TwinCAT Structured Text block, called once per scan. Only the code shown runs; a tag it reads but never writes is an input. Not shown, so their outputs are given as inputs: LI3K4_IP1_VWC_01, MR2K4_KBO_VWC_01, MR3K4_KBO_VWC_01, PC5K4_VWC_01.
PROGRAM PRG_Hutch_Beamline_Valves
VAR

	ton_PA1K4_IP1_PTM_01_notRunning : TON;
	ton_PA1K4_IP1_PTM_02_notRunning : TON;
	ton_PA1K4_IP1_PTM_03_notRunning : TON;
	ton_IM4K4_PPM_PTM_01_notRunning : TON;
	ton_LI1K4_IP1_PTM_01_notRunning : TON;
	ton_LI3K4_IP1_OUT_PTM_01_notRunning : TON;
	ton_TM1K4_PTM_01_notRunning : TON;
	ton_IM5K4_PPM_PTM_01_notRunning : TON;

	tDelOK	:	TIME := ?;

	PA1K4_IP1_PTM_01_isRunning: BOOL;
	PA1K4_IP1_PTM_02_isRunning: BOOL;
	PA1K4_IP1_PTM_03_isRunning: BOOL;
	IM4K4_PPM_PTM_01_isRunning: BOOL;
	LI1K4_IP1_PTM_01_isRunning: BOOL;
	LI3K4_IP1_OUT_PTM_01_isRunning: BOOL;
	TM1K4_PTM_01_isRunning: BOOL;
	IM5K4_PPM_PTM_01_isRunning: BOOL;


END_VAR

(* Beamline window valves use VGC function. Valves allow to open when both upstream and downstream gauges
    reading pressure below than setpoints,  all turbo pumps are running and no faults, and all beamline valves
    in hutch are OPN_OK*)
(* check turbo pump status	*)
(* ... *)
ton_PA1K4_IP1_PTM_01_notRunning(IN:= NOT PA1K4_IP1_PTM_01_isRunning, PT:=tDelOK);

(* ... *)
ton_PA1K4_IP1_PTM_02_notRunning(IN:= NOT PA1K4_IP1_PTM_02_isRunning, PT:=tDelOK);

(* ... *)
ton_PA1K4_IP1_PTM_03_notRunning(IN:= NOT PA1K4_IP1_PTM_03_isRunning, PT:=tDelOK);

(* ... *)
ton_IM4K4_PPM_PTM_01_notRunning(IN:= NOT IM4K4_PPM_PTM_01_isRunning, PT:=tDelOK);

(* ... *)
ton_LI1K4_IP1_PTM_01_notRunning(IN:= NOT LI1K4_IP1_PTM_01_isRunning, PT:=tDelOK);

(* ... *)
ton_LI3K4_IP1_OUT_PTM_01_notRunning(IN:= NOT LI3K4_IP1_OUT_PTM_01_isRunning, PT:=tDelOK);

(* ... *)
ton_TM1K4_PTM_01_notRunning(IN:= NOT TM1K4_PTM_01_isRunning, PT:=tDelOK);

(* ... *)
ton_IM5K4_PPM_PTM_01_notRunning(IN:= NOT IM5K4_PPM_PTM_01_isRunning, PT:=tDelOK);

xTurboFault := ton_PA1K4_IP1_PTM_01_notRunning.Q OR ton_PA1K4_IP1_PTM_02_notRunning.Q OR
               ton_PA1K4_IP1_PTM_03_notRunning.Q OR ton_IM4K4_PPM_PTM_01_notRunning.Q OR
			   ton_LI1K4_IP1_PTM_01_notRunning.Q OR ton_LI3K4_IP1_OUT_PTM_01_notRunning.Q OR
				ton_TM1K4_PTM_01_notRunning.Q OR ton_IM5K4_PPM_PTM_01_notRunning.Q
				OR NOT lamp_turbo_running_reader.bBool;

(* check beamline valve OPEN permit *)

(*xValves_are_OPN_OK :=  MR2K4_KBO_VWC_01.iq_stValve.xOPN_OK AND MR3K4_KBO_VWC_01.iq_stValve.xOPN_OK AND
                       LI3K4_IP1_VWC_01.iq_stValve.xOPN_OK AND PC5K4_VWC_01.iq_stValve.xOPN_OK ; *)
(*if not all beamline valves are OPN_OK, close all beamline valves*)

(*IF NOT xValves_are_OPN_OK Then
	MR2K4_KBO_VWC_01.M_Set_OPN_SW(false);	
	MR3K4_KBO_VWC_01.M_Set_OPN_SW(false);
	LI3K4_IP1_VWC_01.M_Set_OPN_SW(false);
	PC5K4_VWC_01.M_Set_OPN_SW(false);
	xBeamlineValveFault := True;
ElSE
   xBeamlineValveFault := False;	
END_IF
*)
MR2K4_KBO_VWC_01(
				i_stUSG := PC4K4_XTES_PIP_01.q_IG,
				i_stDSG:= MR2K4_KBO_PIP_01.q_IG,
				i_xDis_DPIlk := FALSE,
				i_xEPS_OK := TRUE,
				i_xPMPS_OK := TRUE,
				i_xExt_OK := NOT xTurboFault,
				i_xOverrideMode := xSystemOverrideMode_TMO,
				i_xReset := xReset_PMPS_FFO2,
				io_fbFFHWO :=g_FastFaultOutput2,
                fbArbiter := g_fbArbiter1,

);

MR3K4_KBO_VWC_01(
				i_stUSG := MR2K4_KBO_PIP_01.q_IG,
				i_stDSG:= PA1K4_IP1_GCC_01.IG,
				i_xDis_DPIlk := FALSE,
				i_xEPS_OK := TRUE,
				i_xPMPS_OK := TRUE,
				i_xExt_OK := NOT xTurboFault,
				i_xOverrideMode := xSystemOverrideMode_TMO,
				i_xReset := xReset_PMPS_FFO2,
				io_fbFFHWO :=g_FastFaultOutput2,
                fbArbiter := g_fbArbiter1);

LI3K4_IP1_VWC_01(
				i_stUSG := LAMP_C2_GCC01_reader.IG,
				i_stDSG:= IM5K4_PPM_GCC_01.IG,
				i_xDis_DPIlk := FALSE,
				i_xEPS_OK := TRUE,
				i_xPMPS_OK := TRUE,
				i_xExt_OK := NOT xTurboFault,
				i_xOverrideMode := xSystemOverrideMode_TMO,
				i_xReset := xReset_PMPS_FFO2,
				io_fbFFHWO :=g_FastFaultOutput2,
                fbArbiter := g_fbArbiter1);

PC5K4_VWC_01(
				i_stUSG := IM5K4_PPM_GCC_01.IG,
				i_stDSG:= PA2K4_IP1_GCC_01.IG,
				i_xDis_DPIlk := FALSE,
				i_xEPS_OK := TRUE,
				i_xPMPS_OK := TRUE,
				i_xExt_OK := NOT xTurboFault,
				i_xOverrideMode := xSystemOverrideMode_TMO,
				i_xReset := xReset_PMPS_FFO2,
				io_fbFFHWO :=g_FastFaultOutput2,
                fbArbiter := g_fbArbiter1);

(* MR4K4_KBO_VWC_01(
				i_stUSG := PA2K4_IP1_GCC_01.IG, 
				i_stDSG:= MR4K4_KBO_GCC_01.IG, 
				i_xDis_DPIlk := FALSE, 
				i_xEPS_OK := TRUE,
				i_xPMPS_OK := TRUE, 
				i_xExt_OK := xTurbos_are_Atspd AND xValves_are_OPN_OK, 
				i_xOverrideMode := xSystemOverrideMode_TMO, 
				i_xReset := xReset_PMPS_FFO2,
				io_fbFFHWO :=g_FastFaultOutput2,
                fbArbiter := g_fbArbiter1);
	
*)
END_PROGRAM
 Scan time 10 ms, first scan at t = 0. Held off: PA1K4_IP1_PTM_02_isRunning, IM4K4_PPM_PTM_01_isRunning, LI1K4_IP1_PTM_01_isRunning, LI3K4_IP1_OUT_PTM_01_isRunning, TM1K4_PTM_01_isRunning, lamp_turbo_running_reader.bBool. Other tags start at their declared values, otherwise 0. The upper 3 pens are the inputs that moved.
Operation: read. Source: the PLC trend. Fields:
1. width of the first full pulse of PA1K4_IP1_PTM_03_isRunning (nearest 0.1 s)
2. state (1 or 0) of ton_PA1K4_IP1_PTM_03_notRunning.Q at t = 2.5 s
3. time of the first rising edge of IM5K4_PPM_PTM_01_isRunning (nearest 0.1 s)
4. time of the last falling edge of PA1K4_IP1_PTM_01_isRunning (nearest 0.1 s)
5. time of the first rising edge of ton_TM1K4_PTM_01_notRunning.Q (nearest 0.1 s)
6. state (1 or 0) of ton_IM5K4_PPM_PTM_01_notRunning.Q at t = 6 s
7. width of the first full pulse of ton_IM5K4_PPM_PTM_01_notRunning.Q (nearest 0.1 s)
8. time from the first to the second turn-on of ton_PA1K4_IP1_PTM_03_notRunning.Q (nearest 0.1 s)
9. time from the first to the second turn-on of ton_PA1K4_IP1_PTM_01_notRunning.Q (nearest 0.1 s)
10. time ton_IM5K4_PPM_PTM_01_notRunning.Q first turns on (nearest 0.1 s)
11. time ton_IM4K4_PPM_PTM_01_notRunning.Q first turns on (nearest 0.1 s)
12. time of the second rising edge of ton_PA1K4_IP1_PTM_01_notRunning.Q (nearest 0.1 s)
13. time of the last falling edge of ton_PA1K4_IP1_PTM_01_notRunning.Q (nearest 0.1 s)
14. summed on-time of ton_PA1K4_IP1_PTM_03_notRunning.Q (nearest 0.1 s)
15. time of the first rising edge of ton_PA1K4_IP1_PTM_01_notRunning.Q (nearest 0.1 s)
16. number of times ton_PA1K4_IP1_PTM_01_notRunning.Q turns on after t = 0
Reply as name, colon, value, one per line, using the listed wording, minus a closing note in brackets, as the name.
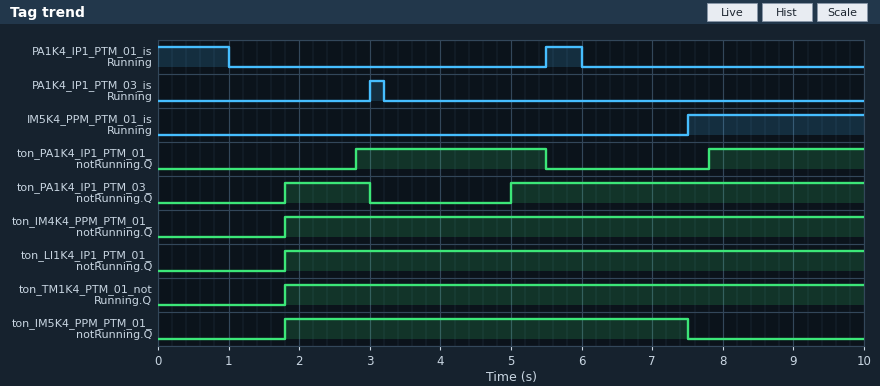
width of the first full pulse of PA1K4_IP1_PTM_03_isRunning: 0.2 s
state (1 or 0) of ton_PA1K4_IP1_PTM_03_notRunning.Q at t = 2.5 s: 1
time of the first rising edge of IM5K4_PPM_PTM_01_isRunning: 7.5 s
time of the last falling edge of PA1K4_IP1_PTM_01_isRunning: 6.0 s
time of the first rising edge of ton_TM1K4_PTM_01_notRunning.Q: 1.8 s
state (1 or 0) of ton_IM5K4_PPM_PTM_01_notRunning.Q at t = 6 s: 1
width of the first full pulse of ton_IM5K4_PPM_PTM_01_notRunning.Q: 5.7 s
time from the first to the second turn-on of ton_PA1K4_IP1_PTM_03_notRunning.Q: 3.2 s
time from the first to the second turn-on of ton_PA1K4_IP1_PTM_01_notRunning.Q: 5.0 s
time ton_IM5K4_PPM_PTM_01_notRunning.Q first turns on: 1.8 s
time ton_IM4K4_PPM_PTM_01_notRunning.Q first turns on: 1.8 s
time of the second rising edge of ton_PA1K4_IP1_PTM_01_notRunning.Q: 7.8 s
time of the last falling edge of ton_PA1K4_IP1_PTM_01_notRunning.Q: 5.5 s
summed on-time of ton_PA1K4_IP1_PTM_03_notRunning.Q: 6.2 s
time of the first rising edge of ton_PA1K4_IP1_PTM_01_notRunning.Q: 2.8 s
number of times ton_PA1K4_IP1_PTM_01_notRunning.Q turns on after t = 0: 2
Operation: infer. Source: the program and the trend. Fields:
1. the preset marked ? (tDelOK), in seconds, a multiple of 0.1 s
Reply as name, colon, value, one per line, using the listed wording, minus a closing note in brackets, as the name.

the preset marked ? (tDelOK), in seconds, a multiple of 0.1 s: 1.8 s
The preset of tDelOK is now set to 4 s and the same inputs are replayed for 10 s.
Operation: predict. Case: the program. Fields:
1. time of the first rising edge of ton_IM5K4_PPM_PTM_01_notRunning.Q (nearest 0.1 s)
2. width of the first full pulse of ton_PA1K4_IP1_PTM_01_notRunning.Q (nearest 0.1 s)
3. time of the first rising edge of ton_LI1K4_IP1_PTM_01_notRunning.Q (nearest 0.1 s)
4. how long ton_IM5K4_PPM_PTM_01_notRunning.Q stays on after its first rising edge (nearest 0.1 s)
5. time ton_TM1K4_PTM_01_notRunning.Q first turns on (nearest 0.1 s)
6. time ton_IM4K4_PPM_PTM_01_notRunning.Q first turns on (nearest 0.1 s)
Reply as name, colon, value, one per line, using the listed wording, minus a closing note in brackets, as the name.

time of the first rising edge of ton_IM5K4_PPM_PTM_01_notRunning.Q: 4.0 s
width of the first full pulse of ton_PA1K4_IP1_PTM_01_notRunning.Q: 0.5 s
time of the first rising edge of ton_LI1K4_IP1_PTM_01_notRunning.Q: 4.0 s
how long ton_IM5K4_PPM_PTM_01_notRunning.Q stays on after its first rising edge: 3.5 s
time ton_TM1K4_PTM_01_notRunning.Q first turns on: 4.0 s
time ton_IM4K4_PPM_PTM_01_notRunning.Q first turns on: 4.0 s
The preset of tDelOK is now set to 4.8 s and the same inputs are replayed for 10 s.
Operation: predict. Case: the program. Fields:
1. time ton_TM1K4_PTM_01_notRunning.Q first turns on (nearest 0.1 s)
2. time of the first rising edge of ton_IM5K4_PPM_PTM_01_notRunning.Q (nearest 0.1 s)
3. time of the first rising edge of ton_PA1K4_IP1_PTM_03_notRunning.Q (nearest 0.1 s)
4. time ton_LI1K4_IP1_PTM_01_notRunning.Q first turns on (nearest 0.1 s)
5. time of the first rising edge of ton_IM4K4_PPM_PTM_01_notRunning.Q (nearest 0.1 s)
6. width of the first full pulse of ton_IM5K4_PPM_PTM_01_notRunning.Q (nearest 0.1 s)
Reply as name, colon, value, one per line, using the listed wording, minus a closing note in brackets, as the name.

time ton_TM1K4_PTM_01_notRunning.Q first turns on: 4.8 s
time of the first rising edge of ton_IM5K4_PPM_PTM_01_notRunning.Q: 4.8 s
time of the first rising edge of ton_PA1K4_IP1_PTM_03_notRunning.Q: 8.0 s
time ton_LI1K4_IP1_PTM_01_notRunning.Q first turns on: 4.8 s
time of the first rising edge of ton_IM4K4_PPM_PTM_01_notRunning.Q: 4.8 s
width of the first full pulse of ton_IM5K4_PPM_PTM_01_notRunning.Q: 2.7 s
